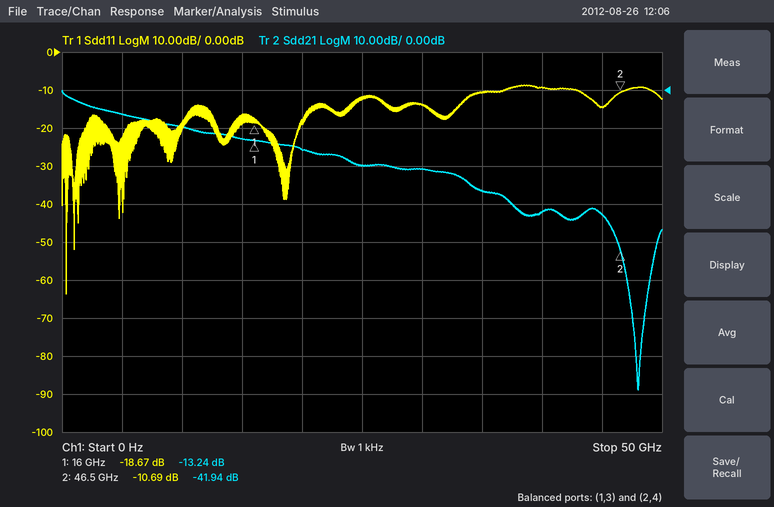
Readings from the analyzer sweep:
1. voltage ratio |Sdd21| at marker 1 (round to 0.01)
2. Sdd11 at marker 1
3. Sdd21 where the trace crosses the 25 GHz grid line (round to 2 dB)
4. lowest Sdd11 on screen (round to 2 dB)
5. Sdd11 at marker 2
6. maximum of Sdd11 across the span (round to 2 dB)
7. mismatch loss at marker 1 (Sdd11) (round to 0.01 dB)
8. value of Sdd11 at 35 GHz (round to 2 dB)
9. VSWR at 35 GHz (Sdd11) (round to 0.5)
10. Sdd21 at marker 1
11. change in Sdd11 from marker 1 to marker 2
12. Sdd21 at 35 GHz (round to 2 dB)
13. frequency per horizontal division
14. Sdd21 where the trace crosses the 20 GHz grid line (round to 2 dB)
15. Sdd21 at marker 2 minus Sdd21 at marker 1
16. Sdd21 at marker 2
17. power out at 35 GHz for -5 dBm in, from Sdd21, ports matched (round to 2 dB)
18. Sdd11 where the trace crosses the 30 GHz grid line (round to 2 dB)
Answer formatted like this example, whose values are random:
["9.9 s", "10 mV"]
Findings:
["0.22", "-18.67 dB", "-20 dB", "-64 dB", "-10.69 dB", "-8 dB", "0.06 dB", "-10 dB", "2.0", "-13.24 dB", "7.98 dB", "-26 dB", "5 GHz", "-16 dB", "-28.70 dB", "-41.94 dB", "-32 dBm", "-14 dB"]
